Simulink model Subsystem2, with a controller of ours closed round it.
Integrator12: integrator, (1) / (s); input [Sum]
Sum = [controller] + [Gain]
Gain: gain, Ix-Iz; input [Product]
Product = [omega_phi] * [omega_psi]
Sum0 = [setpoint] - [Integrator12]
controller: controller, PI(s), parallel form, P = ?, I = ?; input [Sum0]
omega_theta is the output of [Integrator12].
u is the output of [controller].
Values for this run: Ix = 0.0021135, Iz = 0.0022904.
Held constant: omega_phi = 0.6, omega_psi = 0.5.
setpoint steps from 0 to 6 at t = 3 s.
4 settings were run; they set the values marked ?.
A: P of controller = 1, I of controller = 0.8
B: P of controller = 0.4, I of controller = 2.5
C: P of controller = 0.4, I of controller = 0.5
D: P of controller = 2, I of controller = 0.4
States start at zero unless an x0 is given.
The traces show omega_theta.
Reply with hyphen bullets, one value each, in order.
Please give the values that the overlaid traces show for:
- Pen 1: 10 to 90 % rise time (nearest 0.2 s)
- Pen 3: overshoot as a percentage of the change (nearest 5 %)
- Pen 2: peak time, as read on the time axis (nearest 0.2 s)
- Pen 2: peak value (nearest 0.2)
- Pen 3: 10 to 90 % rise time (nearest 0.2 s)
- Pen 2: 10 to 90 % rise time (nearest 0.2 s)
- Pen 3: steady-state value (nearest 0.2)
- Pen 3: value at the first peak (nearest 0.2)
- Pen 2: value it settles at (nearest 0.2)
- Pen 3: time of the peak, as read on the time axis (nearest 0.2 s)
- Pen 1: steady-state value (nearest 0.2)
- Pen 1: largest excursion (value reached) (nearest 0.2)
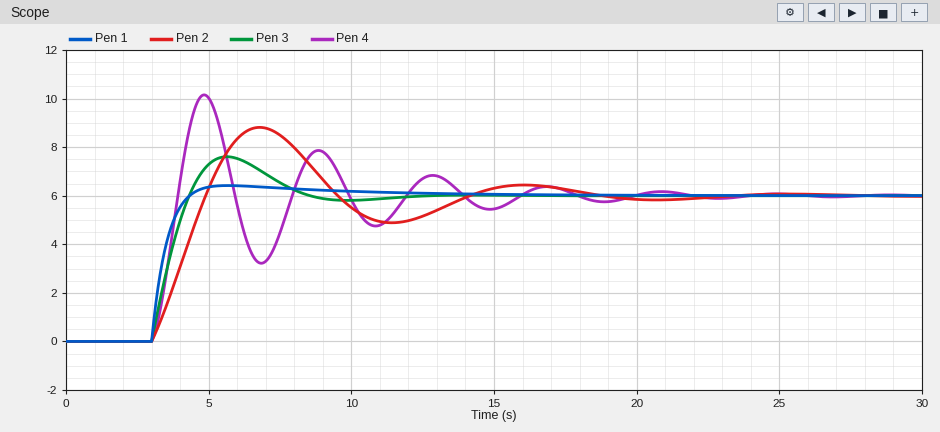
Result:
- 0.8 s
- 25 %
- 6.8 s
- 8.8
- 1.0 s
- 1.4 s
- 6.0
- 7.6
- 6.0
- 5.6 s
- 6.0
- 6.4
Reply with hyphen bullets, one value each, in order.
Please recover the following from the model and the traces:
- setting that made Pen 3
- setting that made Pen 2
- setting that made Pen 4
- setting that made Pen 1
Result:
- A
- C
- B
- D
